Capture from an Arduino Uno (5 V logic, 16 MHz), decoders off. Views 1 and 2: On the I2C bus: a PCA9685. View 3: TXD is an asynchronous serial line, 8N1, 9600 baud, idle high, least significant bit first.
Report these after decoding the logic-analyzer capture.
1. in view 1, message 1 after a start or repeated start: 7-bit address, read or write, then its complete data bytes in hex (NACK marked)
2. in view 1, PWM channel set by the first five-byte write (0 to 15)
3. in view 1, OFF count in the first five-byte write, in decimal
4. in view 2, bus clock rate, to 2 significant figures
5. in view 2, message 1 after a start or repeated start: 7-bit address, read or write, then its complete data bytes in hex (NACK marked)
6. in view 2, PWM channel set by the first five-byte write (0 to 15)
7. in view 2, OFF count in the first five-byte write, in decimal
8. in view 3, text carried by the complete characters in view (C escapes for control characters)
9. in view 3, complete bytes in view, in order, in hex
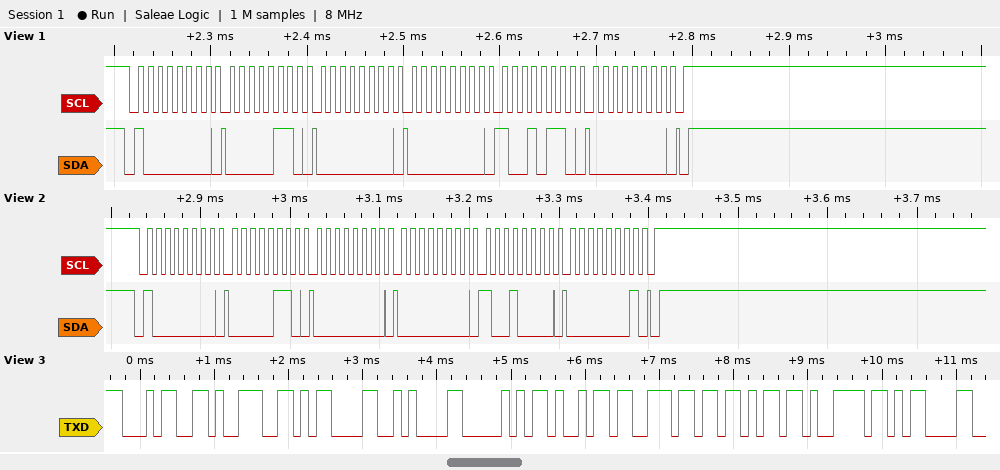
0x40 write: 06 00 00 96 00
0
150
100 kHz
0x40 write: 06 00 00 90 01
0
400
"49\r\nPinky\r"
34 39 0D 0A 50 69 6E 6B 79 0D
